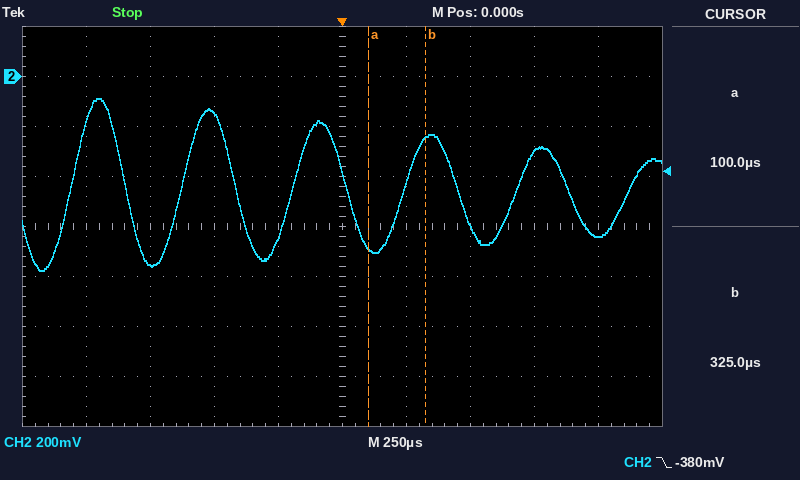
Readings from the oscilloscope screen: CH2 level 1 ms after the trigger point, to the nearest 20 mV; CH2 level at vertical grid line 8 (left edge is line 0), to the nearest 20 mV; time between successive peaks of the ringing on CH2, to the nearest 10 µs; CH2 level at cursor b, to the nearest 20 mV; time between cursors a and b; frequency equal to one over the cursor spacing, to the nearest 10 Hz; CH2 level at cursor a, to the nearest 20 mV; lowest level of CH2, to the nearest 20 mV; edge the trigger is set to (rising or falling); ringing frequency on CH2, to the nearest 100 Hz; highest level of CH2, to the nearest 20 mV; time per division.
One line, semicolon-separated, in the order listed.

-640 mV; -300 mV; 430 µs; -240 mV; 225 µs; 4.44 kHz; -680 mV; -780 mV; falling; 2.3 kHz; -80 mV; 250 µs
